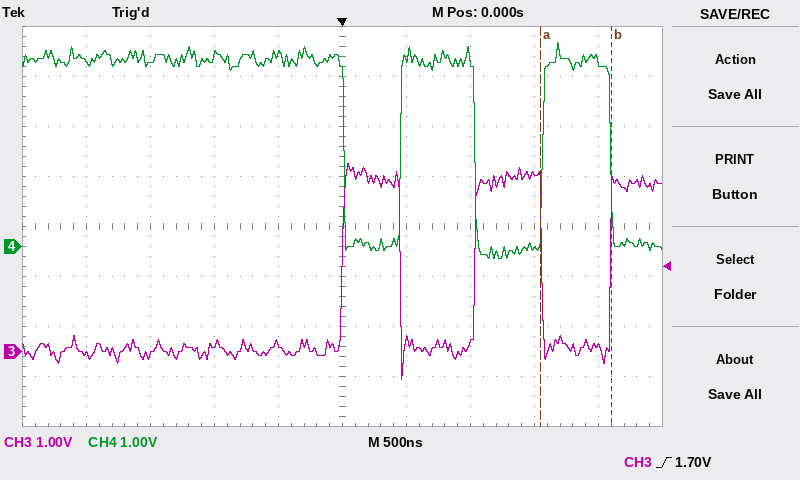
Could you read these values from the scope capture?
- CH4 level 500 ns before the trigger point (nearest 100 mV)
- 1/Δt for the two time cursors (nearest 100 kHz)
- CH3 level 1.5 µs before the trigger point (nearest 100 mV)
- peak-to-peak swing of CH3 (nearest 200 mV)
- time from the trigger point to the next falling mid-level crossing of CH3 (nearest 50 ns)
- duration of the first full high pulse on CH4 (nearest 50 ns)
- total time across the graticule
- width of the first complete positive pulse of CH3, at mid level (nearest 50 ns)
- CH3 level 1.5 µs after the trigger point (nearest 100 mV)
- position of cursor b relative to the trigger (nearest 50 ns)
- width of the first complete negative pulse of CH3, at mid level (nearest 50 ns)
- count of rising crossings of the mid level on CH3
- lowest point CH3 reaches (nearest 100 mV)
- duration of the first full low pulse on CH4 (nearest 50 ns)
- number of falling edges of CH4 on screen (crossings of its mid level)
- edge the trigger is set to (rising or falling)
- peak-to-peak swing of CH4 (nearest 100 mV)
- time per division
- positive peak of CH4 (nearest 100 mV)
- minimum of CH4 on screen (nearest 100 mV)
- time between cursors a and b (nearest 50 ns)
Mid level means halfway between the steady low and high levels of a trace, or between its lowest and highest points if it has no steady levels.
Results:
3.8 V
1.8 MHz
-100 mV
4.4 V
450 ns
600 ns
5 µs
450 ns
3.6 V
+2.10 µs
600 ns
3
-600 mV
450 ns
3
rising
4.3 V
500 ns
4.1 V
-200 mV
550 ns
